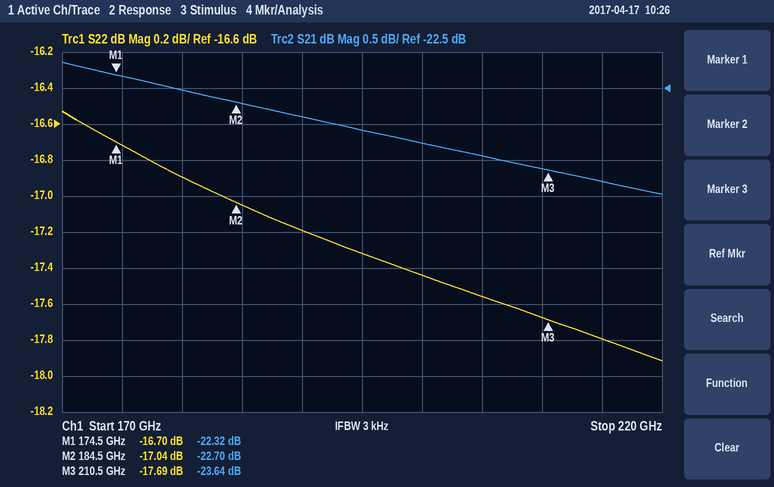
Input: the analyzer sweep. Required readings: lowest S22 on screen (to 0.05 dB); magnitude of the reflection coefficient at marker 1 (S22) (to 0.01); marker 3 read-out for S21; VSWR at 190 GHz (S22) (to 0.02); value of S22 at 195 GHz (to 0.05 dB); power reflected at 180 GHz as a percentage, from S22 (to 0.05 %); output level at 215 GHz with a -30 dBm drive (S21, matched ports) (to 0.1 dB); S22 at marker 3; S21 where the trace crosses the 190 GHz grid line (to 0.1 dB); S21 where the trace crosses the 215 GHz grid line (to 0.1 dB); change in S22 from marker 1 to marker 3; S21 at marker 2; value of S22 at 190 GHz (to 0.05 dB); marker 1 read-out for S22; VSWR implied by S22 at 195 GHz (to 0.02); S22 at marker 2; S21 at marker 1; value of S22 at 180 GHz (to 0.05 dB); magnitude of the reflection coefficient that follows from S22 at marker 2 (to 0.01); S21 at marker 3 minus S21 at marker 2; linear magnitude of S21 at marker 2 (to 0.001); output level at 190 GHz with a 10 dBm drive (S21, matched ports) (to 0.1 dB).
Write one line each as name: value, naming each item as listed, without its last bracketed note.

lowest S22 on screen: -17.90 dB
magnitude of the reflection coefficient at marker 1 (S22): 0.15
marker 3 read-out for S21: -23.64 dB
VSWR at 190 GHz (S22): 1.32
value of S22 at 195 GHz: -17.30 dB
power reflected at 180 GHz as a percentage, from S22: 2.05 %
output level at 215 GHz with a -30 dBm drive (S21, matched ports): -53.8 dBm
S22 at marker 3: -17.69 dB
S21 where the trace crosses the 190 GHz grid line: -22.9 dB
S21 where the trace crosses the 215 GHz grid line: -23.8 dB
change in S22 from marker 1 to marker 3: -0.99 dB
S21 at marker 2: -22.70 dB
value of S22 at 190 GHz: -17.20 dB
marker 1 read-out for S22: -16.70 dB
VSWR implied by S22 at 195 GHz: 1.32
S22 at marker 2: -17.04 dB
S21 at marker 1: -22.32 dB
value of S22 at 180 GHz: -16.90 dB
magnitude of the reflection coefficient that follows from S22 at marker 2: 0.14
S21 at marker 3 minus S21 at marker 2: -0.94 dB
linear magnitude of S21 at marker 2: 0.073
output level at 190 GHz with a 10 dBm drive (S21, matched ports): -12.9 dBm
